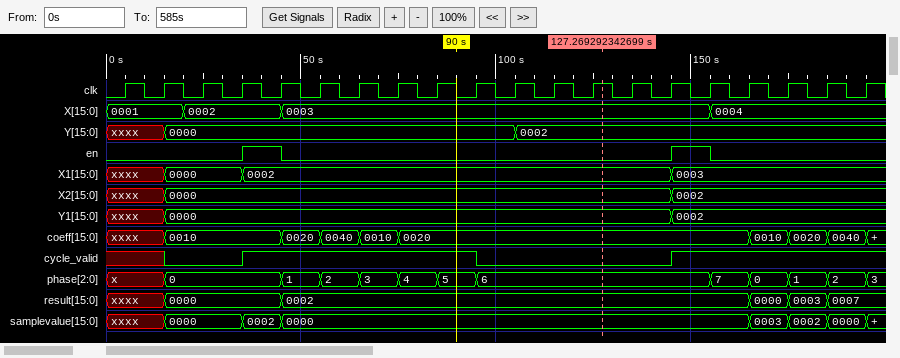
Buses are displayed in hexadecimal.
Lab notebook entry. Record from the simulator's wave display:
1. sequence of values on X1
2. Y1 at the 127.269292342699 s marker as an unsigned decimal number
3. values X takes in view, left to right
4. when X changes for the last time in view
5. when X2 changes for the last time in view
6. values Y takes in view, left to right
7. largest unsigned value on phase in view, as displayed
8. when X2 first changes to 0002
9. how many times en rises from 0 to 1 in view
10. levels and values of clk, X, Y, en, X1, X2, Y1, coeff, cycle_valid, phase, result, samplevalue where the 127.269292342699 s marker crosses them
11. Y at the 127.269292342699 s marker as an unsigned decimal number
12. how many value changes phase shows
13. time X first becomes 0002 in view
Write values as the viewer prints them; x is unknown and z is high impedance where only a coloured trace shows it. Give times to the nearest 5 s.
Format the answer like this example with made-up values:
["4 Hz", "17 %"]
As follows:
["xxxx, 0000, 0002, 0003", "0", "0001, 0002, 0003, 0004", "155 s", "145 s", "xxxx, 0000, 0002", "7", "145 s", "2", "clk=1, X=0003, Y=0002, en=0, X1=0002, X2=0000, Y1=0000, coeff=0020, cycle_valid=0, phase=6, result=0002, samplevalue=0000", "2", "12", "20 s"]
